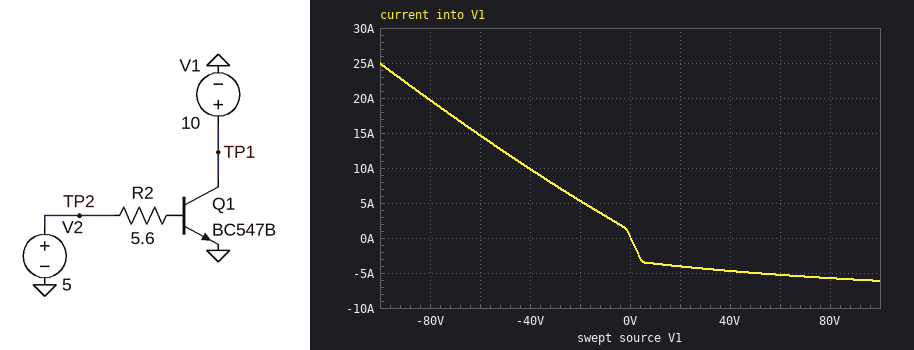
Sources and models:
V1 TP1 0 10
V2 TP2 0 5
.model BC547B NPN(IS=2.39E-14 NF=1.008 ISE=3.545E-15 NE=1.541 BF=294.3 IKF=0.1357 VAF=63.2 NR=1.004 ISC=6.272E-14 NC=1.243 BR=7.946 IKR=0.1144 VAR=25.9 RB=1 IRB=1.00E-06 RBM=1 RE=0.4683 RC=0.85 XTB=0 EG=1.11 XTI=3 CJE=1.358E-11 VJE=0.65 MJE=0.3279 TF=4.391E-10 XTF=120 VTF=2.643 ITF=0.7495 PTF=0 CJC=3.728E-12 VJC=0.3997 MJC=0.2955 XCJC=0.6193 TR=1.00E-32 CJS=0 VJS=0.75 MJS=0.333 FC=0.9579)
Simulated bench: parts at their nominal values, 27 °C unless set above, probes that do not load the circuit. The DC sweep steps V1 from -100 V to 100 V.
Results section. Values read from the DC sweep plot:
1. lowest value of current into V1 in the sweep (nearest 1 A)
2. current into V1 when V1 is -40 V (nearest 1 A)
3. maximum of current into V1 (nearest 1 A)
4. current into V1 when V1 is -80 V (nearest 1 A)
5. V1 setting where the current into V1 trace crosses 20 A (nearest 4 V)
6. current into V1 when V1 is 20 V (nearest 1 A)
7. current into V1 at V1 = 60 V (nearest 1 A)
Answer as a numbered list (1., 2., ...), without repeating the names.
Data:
1. -6 A
2. 10 A
3. 25 A
4. 20 A
5. -80 V
6. -4 A
7. -5 A
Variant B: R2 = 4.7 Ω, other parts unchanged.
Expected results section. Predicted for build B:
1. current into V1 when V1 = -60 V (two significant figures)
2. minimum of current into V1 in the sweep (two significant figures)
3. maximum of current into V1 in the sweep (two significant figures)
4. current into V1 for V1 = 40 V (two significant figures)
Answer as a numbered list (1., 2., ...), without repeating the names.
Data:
1. 16 A
2. -6.3 A
3. 27 A
4. -4.9 A
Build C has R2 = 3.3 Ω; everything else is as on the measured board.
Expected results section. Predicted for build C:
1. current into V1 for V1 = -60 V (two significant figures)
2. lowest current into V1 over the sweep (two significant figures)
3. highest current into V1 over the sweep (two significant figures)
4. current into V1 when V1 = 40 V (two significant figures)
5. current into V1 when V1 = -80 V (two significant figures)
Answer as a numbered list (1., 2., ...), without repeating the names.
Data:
1. 19 A
2. -6.6 A
3. 32 A
4. -5.3 A
5. 25 A
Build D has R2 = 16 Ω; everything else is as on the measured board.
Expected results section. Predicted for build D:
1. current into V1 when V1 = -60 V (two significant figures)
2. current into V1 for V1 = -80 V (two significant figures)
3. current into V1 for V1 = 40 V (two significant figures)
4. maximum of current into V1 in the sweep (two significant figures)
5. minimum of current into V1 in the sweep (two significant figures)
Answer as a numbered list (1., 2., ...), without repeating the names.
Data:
1. 8.2 A
2. 11 A
3. -3.5 A
4. 14 A
5. -4.8 A
